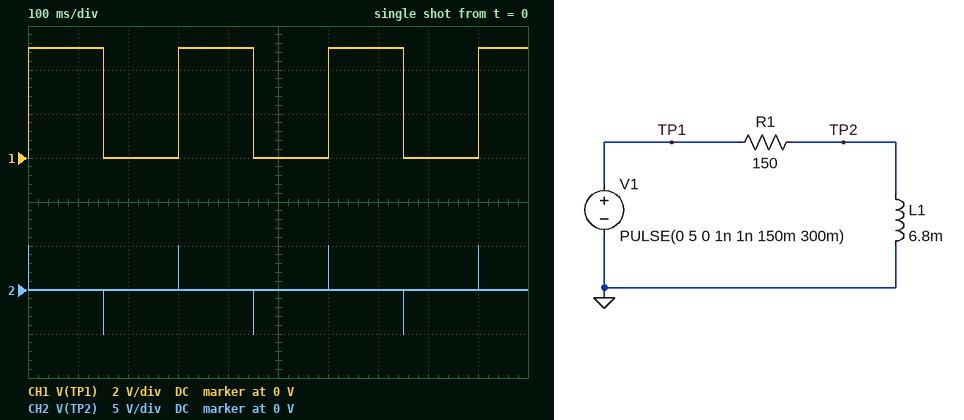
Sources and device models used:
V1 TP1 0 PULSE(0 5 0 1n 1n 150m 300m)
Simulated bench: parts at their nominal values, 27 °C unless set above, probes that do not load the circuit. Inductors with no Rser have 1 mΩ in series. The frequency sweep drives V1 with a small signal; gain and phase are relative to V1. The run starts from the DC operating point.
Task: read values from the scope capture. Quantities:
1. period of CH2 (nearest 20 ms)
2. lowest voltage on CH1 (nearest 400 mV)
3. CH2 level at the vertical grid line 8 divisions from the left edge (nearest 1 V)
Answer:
300 ms
0 V
0 V
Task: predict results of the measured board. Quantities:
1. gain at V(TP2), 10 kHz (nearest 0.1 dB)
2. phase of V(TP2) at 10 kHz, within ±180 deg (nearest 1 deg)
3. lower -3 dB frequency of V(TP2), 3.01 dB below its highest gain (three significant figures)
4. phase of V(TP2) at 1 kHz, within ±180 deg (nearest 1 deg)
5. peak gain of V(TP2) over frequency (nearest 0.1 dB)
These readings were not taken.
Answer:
-0.5 dB
19 deg
3.51 kHz
74 deg
0 dB
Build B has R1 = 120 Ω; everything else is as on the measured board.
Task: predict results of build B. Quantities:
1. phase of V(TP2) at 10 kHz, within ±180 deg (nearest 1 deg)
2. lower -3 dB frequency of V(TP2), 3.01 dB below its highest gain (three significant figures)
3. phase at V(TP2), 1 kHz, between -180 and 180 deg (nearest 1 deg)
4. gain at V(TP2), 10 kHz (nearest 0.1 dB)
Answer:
16 deg
2.81 kHz
70 deg
-0.3 dB
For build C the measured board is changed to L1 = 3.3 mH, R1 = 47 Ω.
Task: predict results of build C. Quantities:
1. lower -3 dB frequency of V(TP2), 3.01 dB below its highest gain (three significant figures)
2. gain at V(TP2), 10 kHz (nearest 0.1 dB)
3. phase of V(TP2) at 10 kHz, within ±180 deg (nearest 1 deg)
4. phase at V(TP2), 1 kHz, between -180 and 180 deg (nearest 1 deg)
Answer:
2.27 kHz
-0.2 dB
13 deg
66 deg
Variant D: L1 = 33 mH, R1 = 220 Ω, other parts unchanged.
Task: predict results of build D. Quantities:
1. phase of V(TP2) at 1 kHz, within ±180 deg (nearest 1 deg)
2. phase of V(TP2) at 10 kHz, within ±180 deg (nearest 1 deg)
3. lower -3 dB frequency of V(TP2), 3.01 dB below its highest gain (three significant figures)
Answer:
47 deg
6 deg
1.06 kHz
